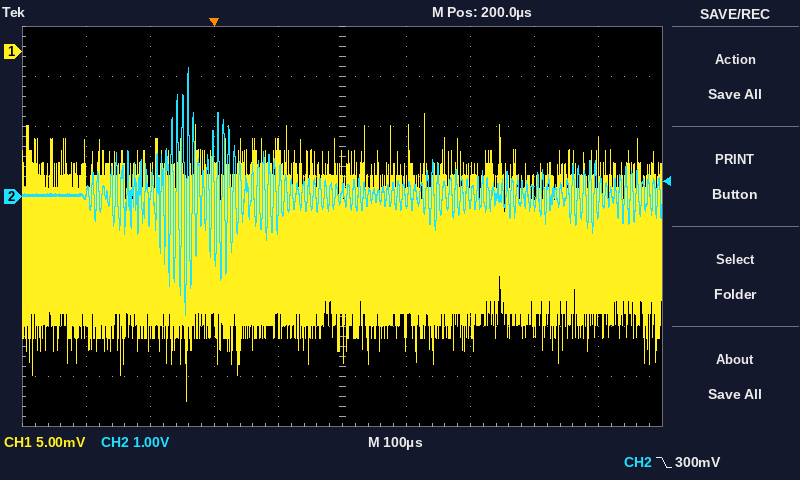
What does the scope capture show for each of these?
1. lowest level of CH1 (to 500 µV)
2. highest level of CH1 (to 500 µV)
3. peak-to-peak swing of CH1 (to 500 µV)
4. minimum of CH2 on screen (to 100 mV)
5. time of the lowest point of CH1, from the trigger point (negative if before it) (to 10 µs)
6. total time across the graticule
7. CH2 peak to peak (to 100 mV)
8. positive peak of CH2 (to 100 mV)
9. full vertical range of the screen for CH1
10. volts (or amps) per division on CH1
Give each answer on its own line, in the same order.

-35.0 mV
-6.0 mV
29.0 mV
-2.4 V
-40 µs
1 ms
5.0 V
2.6 V
40 mV
5 mV
